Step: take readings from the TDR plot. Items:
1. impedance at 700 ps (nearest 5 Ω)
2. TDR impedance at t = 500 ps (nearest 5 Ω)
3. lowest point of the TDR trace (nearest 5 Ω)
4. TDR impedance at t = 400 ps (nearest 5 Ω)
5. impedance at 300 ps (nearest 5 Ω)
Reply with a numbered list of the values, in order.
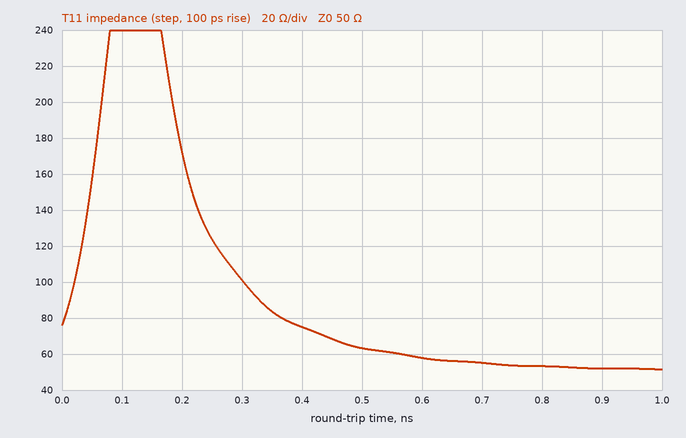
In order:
1. 55 Ω
2. 65 Ω
3. 50 Ω
4. 75 Ω
5. 100 Ω
